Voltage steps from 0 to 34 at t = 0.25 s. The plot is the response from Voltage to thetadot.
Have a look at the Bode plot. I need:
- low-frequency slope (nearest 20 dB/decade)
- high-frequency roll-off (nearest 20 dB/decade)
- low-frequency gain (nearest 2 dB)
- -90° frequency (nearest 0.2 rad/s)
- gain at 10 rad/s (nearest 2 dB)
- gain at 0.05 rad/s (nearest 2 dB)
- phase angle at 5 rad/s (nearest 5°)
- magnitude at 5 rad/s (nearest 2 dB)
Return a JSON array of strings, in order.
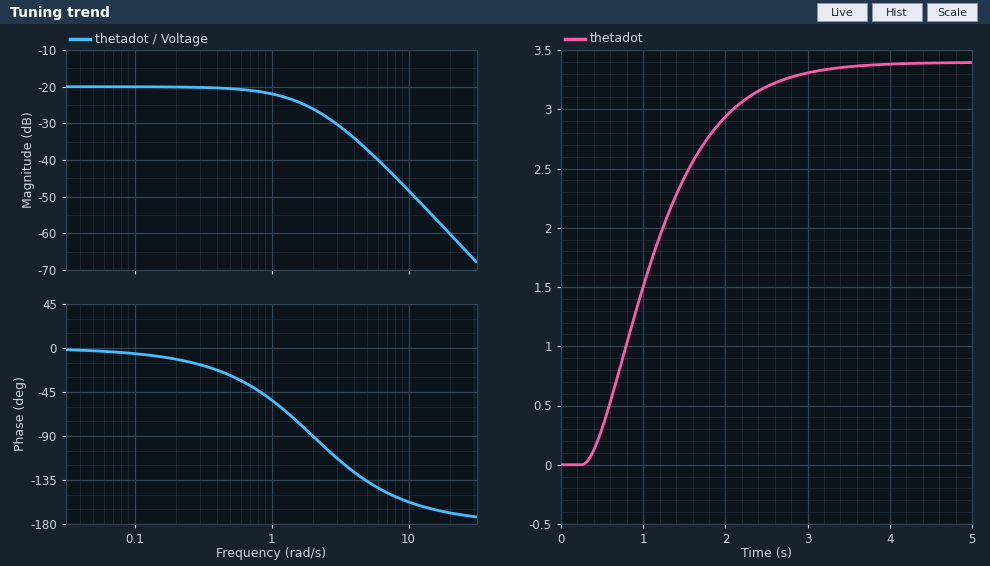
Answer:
["0 dB/decade", "-40 dB/decade", "-20 dB", "2.0 rad/s", "-48 dB", "-20 dB", "-135°", "-38 dB"]
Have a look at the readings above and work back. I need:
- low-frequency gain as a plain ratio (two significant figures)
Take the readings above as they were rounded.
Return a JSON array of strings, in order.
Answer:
["0.10"]
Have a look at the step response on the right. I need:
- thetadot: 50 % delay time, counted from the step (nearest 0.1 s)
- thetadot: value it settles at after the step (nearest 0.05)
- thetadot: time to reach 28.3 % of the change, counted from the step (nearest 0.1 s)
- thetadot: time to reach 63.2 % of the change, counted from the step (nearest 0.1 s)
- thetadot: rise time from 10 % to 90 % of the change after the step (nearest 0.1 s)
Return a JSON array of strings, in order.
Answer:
["0.8 s", "3.40", "0.5 s", "1.1 s", "1.7 s"]
